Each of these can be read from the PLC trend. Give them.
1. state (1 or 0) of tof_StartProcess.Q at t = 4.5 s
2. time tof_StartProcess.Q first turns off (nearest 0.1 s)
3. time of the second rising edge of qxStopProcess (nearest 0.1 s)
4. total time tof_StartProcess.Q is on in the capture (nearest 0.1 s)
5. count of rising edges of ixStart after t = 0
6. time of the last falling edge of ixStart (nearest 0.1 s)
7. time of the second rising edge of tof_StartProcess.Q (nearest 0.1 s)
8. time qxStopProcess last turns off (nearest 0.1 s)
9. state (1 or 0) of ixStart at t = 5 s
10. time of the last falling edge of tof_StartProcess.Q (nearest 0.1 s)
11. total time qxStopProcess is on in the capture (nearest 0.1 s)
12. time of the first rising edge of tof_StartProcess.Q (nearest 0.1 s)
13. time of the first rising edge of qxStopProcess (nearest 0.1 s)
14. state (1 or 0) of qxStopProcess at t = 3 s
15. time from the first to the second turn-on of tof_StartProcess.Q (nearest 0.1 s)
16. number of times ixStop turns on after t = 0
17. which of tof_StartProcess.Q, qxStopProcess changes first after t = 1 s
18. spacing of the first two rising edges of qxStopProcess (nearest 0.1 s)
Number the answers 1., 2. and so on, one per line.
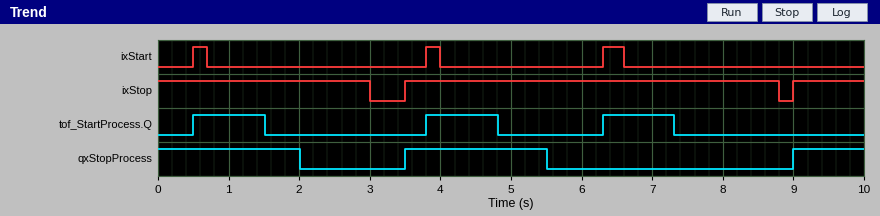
1. 1
2. 1.5 s
3. 9.0 s
4. 3.0 s
5. 3
6. 6.6 s
7. 3.8 s
8. 5.5 s
9. 0
10. 7.3 s
11. 5.0 s
12. 0.5 s
13. 3.5 s
14. 0
15. 3.3 s
16. 2
17. tof_StartProcess.Q
18. 5.5 s
